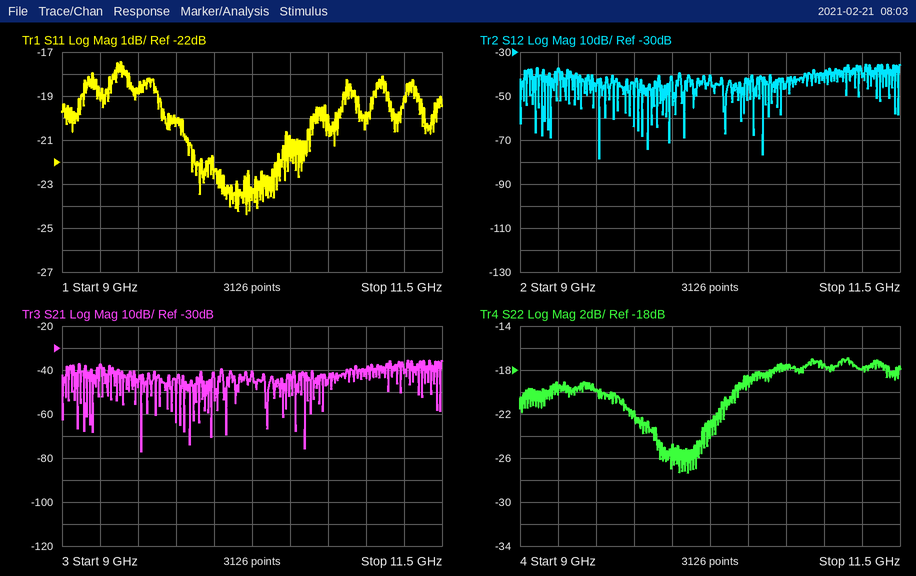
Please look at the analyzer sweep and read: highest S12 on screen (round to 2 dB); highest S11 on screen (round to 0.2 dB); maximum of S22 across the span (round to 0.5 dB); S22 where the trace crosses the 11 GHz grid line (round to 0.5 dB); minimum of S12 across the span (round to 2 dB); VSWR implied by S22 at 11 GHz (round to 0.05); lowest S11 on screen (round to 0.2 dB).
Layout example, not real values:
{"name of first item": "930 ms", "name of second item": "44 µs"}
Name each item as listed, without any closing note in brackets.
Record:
{"highest S12 on screen": "-36 dB", "highest S11 on screen": "-17.4 dB", "maximum of S22 across the span": "-17.0 dB", "S22 where the trace crosses the 11 GHz grid line": "-17.5 dB", "minimum of S12 across the span": "-78 dB", "VSWR implied by S22 at 11 GHz": "1.30", "lowest S11 on screen": "-24.4 dB"}
